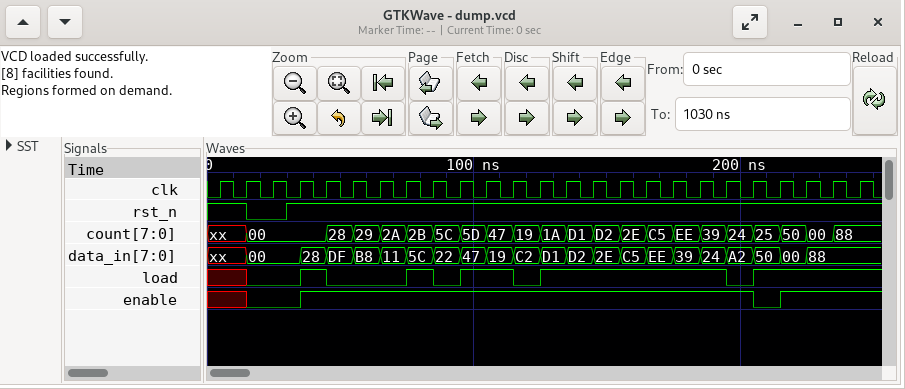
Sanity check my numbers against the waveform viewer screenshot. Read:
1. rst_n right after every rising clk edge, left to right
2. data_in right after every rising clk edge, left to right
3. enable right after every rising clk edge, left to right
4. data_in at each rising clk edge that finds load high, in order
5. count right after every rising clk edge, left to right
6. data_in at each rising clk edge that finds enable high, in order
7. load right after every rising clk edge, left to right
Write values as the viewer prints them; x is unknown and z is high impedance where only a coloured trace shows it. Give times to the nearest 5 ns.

1 0 0 1 1 1 1 1 1 1 1 1 1 1 1 1 1 1 1 1 1 1 1 1 1
xx, 00, 00, 28, DF, B8, 11, 5C, 22, 47, 19, C2, D1, D2, 2E, C5, EE, 39, 24, A2, 50, 00, 88, 88, 88
x 0 0 1 1 1 1 1 1 1 1 1 1 1 1 1 1 1 1 1 0 1 1 1 1
28, 5C, 47, 19, D1, D2, 2E, C5, EE, 39, 24, 50, 00, 88, 88
xx, 00, 00, 00, 28, 29, 2A, 2B, 5C, 5D, 47, 19, 1A, D1, D2, 2E, C5, EE, 39, 24, 25, 50, 00, 88, 88
28, DF, B8, 11, 5C, 22, 47, 19, C2, D1, D2, 2E, C5, EE, 39, 24, A2, 00, 88, 88
x 0 0 1 0 0 0 1 0 1 1 0 1 1 1 1 1 1 1 0 1 1 1 1 1
